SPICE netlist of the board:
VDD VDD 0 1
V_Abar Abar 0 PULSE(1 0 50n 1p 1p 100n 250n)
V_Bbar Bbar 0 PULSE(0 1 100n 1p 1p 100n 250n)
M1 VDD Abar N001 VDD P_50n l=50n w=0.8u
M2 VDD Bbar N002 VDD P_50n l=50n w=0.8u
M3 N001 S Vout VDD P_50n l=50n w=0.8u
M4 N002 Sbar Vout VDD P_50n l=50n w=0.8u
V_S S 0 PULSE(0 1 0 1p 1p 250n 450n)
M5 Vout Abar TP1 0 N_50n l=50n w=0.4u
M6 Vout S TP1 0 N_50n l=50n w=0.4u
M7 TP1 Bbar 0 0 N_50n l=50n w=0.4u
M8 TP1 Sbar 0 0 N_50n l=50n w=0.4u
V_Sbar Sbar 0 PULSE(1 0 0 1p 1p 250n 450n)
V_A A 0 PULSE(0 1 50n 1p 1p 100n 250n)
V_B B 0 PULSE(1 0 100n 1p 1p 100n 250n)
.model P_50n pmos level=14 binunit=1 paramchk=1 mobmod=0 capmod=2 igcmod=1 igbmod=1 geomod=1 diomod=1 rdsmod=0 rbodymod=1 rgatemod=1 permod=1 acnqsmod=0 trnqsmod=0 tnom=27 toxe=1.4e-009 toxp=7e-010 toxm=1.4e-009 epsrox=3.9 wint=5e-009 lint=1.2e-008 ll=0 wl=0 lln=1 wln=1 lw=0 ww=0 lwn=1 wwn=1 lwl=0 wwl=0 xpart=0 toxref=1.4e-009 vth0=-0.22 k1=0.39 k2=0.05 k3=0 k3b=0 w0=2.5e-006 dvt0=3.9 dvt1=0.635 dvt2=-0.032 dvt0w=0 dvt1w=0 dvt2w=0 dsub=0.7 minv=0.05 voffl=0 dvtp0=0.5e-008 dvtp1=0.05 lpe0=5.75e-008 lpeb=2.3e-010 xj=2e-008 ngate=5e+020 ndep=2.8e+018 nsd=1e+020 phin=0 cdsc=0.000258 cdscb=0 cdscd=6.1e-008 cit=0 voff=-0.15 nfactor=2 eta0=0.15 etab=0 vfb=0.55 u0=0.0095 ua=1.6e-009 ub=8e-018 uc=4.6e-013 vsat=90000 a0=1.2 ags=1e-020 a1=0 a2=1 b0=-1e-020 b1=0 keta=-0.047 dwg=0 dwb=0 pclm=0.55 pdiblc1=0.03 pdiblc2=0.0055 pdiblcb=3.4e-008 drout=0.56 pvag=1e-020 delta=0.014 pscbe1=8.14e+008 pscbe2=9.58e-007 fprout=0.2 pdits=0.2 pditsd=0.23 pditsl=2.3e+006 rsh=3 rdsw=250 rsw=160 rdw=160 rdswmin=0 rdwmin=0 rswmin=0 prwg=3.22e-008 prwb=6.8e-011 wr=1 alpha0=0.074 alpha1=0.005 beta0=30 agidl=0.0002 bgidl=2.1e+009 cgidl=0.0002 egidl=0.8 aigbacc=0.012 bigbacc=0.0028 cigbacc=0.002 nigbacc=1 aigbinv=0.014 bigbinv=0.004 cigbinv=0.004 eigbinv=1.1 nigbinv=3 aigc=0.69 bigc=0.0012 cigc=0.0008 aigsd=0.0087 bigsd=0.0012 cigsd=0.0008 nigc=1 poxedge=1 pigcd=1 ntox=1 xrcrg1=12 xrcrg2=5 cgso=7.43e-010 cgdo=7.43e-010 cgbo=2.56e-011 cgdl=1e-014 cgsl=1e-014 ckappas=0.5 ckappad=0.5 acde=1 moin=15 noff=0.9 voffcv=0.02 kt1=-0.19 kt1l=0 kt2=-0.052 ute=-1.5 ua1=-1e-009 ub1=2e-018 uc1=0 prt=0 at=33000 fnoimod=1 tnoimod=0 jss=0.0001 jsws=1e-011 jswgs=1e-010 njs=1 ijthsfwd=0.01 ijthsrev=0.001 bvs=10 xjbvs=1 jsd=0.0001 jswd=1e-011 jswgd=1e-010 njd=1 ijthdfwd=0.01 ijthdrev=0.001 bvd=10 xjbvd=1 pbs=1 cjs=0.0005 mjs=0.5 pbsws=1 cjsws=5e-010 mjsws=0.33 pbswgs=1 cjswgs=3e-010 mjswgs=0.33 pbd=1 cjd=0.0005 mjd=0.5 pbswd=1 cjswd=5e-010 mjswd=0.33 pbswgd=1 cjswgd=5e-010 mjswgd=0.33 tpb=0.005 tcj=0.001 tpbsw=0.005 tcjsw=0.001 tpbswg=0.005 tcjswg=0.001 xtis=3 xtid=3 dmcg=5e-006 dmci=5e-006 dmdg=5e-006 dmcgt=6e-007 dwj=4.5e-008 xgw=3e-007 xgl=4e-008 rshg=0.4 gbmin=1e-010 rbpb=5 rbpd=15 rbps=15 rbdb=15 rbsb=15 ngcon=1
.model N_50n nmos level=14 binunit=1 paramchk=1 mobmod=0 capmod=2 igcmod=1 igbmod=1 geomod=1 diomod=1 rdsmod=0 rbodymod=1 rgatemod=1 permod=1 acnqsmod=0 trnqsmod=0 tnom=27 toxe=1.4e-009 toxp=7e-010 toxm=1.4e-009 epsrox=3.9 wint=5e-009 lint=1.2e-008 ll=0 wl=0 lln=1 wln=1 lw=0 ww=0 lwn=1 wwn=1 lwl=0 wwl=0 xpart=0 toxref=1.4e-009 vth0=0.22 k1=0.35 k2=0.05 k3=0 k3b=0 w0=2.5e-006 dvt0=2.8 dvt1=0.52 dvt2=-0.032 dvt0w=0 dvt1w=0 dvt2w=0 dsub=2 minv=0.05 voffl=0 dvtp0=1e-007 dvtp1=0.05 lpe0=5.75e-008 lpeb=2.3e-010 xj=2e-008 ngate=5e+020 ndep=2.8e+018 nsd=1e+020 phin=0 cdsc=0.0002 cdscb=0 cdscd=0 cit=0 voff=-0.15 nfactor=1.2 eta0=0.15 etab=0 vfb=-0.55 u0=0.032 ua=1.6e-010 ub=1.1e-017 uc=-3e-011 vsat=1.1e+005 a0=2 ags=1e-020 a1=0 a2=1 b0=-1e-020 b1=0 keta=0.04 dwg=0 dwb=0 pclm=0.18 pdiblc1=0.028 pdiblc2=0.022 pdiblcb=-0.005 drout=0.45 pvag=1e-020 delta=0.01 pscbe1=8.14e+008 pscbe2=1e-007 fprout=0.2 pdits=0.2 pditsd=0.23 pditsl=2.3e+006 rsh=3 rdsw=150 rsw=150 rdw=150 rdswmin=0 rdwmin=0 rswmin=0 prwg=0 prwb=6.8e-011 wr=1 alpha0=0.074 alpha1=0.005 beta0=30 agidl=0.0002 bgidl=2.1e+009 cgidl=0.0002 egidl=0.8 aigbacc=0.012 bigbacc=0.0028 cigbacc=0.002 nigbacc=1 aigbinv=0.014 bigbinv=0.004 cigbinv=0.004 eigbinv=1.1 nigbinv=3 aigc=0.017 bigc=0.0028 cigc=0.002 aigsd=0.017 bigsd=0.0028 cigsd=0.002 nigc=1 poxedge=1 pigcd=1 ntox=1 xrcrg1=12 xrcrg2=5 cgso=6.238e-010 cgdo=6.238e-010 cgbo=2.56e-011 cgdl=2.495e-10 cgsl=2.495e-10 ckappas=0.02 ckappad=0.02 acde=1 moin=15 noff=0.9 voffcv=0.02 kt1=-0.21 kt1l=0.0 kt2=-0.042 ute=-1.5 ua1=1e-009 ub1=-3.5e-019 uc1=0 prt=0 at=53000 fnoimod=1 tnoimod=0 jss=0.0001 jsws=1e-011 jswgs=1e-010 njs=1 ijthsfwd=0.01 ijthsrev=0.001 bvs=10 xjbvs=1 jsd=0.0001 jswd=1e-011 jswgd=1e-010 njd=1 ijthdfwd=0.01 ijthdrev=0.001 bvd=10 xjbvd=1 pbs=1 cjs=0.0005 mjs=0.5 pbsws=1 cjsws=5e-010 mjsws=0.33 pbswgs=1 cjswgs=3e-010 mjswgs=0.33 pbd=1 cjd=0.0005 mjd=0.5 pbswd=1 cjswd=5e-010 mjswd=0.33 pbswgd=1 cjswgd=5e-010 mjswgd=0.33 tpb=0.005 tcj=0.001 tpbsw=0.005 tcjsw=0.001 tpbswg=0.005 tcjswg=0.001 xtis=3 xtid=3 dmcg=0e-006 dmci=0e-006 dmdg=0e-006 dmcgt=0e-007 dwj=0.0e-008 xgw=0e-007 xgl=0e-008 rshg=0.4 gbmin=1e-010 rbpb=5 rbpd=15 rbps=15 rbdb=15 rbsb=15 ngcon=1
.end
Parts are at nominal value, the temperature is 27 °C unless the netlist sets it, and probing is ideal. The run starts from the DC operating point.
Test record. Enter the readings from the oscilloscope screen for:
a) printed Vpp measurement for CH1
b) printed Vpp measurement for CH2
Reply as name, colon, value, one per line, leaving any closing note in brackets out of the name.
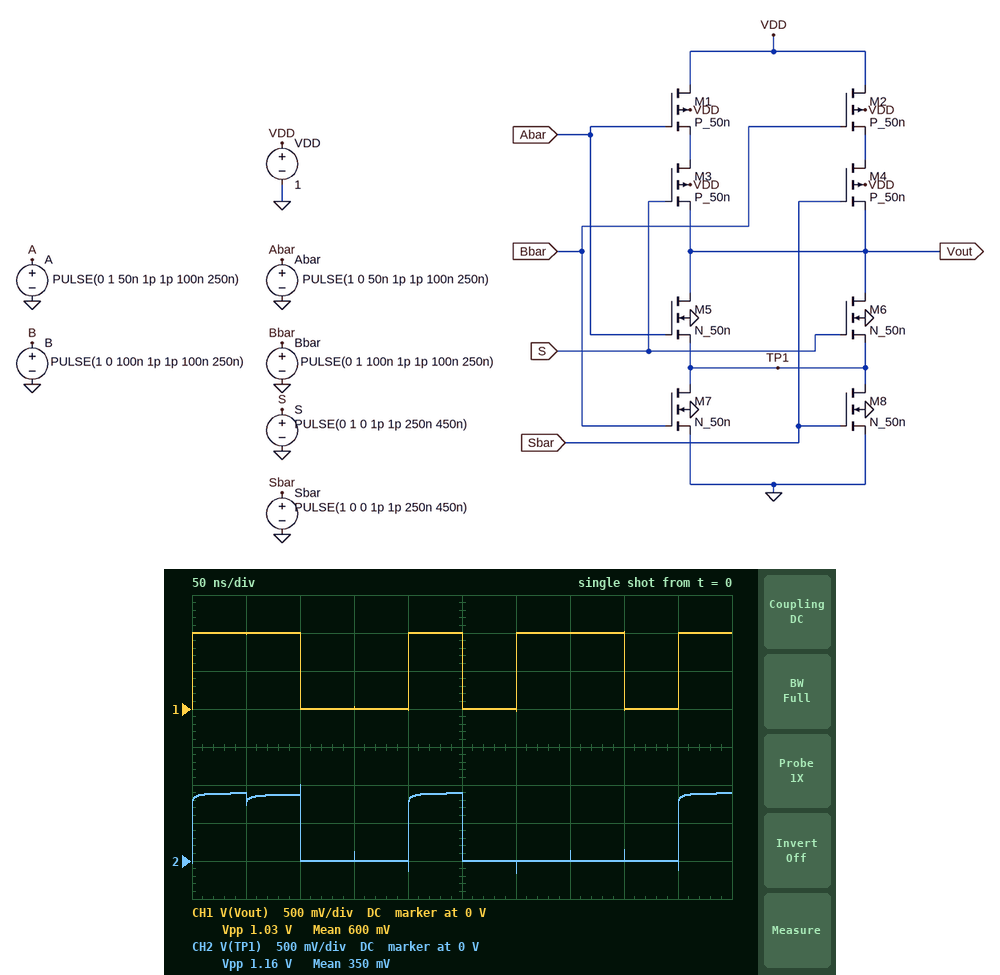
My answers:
printed Vpp measurement for CH1: 1.03 V
printed Vpp measurement for CH2: 1.16 V
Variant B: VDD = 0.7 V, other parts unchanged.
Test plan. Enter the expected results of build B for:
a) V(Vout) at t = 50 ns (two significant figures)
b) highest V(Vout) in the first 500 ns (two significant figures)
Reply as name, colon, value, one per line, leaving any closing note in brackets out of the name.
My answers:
V(Vout) at t = 50 ns: 700 mV
highest V(Vout) in the first 500 ns: 710 mV
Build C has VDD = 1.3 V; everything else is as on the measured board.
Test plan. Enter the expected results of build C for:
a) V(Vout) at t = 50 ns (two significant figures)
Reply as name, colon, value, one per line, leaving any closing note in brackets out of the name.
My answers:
V(Vout) at t = 50 ns: 1.3 V
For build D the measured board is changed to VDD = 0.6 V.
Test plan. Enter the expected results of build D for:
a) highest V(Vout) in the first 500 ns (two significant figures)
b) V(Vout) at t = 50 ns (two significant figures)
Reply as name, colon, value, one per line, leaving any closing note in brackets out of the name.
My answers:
highest V(Vout) in the first 500 ns: 610 mV
V(Vout) at t = 50 ns: 600 mV
